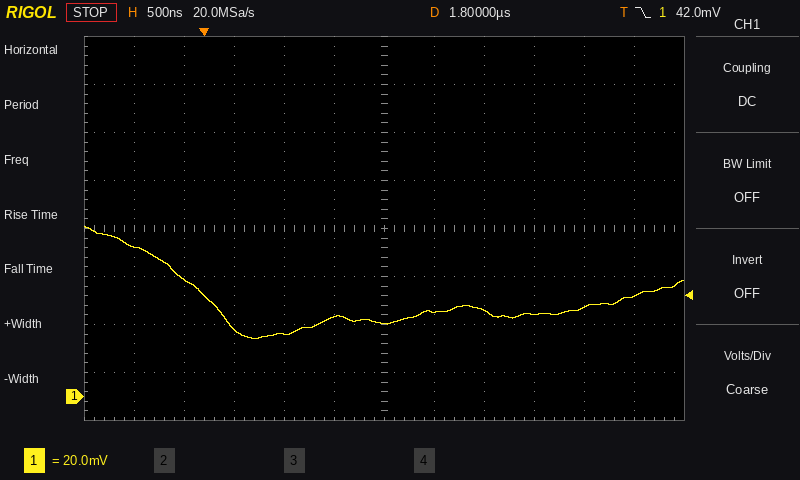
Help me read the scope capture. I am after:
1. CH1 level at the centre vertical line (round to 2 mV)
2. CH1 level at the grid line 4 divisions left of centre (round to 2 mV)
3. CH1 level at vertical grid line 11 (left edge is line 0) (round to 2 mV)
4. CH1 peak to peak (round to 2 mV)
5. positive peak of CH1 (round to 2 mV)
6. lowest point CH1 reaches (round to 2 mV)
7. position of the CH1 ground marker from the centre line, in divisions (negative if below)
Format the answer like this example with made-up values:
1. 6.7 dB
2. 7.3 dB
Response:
1. 30 mV
2. 48 mV
3. 42 mV
4. 46 mV
5. 70 mV
6. 24 mV
7. -3.5 div
